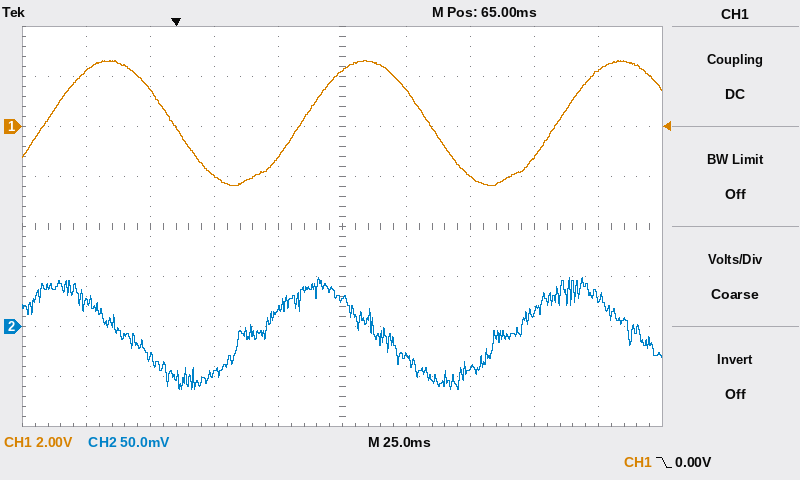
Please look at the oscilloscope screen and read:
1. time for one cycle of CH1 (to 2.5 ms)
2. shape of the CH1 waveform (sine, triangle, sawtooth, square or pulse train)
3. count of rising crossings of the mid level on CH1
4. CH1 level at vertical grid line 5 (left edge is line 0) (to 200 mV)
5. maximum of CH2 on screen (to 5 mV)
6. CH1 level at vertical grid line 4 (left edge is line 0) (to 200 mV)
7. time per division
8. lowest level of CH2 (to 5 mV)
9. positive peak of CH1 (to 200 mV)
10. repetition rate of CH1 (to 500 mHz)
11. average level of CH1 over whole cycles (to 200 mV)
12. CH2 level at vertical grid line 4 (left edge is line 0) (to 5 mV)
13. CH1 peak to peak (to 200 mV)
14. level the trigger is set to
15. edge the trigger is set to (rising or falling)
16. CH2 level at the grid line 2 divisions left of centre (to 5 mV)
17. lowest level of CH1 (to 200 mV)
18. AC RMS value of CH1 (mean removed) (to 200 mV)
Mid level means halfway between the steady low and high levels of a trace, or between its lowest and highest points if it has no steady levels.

100.0 ms
sine
3
2.2 V
50 mV
-1.2 V
25 ms
-65 mV
2.6 V
10.0 Hz
200 mV
15 mV
5.0 V
0.00 V
falling
-45 mV
-2.4 V
1.8 V
